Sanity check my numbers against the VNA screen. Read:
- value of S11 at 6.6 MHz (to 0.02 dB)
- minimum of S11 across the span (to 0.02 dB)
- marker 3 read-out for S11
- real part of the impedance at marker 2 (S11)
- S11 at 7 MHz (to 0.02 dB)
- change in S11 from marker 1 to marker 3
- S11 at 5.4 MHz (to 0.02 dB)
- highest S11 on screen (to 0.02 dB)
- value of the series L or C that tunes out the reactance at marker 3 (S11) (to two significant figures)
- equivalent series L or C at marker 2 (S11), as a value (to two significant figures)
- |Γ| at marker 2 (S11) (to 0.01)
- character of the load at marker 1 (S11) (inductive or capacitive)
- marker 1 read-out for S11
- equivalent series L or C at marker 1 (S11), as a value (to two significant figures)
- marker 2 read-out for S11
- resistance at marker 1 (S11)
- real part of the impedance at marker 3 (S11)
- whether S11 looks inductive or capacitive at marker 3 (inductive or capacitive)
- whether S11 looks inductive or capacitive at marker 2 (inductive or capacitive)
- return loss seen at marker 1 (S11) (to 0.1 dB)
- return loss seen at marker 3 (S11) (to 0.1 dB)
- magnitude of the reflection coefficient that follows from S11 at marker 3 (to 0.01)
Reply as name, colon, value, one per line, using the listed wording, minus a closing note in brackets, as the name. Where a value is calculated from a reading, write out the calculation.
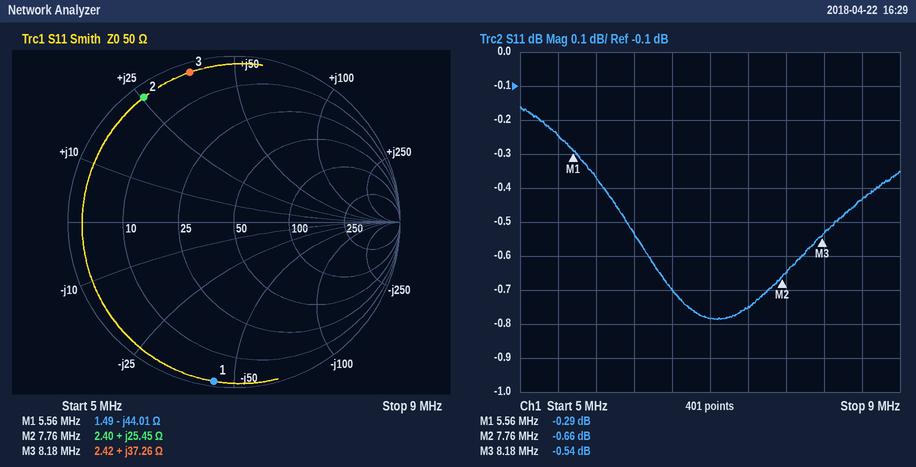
value of S11 at 6.6 MHz: -0.70 dB
minimum of S11 across the span: -0.78 dB
marker 3 read-out for S11: -0.54 dB
real part of the impedance at marker 2: 2.40 Ω
S11 at 7 MHz: -0.78 dB
change in S11 from marker 1 to marker 3: -0.54 − (-0.29) = -0.25 dB
S11 at 5.4 MHz: -0.24 dB
highest S11 on screen: -0.16 dB
value of the series L or C that tunes out the reactance at marker 3 (S11): C = 1/(2π × 8.18 MHz × 37.26 Ω) ≈ 522 pF, so 520 pF to two significant figures
equivalent series L or C at marker 2 (S11), as a value: L = 25.45 Ω/(2π × 7.76 MHz) ≈ 522 nH, so 520 nH to two significant figures
|Γ| at marker 2 (S11): 0.93
character of the load at marker 1 (S11): capacitive
marker 1 read-out for S11: -0.29 dB
equivalent series L or C at marker 1 (S11), as a value: C = 1/(2π × 5.56 MHz × 44.01 Ω) ≈ 650 pF
marker 2 read-out for S11: -0.66 dB
resistance at marker 1: 1.49 Ω
real part of the impedance at marker 3: 2.42 Ω
whether S11 looks inductive or capacitive at marker 3: inductive
whether S11 looks inductive or capacitive at marker 2: inductive
return loss seen at marker 1 (S11): 0.3 dB
return loss seen at marker 3 (S11): 0.5 dB
magnitude of the reflection coefficient that follows from S11 at marker 3: 10^(-0.54/20) ≈ 0.94
